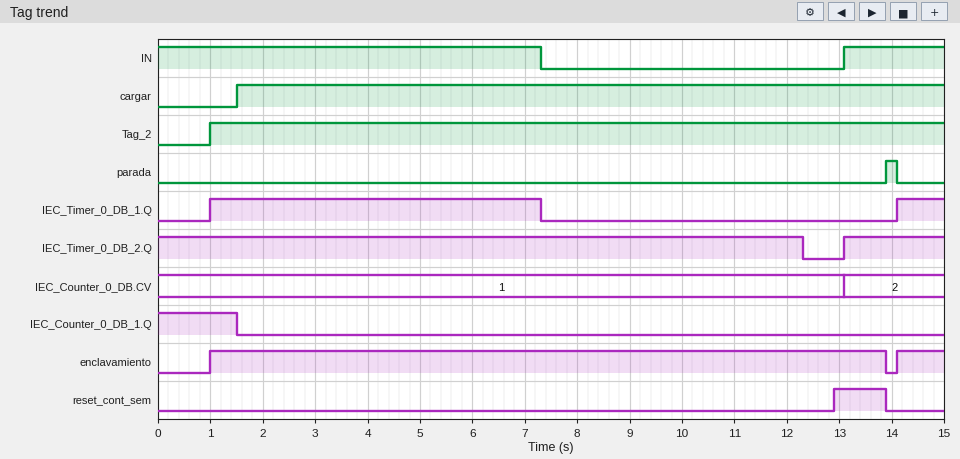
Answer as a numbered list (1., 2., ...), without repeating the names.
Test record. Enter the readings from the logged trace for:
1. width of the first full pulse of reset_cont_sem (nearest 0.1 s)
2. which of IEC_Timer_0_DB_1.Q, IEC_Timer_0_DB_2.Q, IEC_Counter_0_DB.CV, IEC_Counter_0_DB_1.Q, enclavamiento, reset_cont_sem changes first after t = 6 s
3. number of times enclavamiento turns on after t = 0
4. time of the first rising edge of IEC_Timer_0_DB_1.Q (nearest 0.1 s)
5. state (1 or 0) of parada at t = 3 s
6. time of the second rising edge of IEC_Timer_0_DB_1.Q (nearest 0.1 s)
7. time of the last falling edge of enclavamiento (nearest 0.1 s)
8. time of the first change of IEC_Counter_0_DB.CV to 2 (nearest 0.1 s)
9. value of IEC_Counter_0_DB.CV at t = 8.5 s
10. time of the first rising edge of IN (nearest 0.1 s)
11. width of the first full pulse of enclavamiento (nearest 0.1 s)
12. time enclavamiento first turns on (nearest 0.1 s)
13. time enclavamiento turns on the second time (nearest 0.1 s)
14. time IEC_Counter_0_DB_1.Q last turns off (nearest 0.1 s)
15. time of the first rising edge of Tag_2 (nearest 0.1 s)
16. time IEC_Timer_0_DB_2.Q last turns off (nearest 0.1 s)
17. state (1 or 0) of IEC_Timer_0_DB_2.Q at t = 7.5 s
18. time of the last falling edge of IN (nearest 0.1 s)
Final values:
1. 1.0 s
2. IEC_Timer_0_DB_1.Q
3. 2
4. 1.0 s
5. 0
6. 14.1 s
7. 13.9 s
8. 13.1 s
9. 1
10. 13.1 s
11. 12.9 s
12. 1.0 s
13. 14.1 s
14. 1.5 s
15. 1.0 s
16. 12.3 s
17. 1
18. 7.3 s
